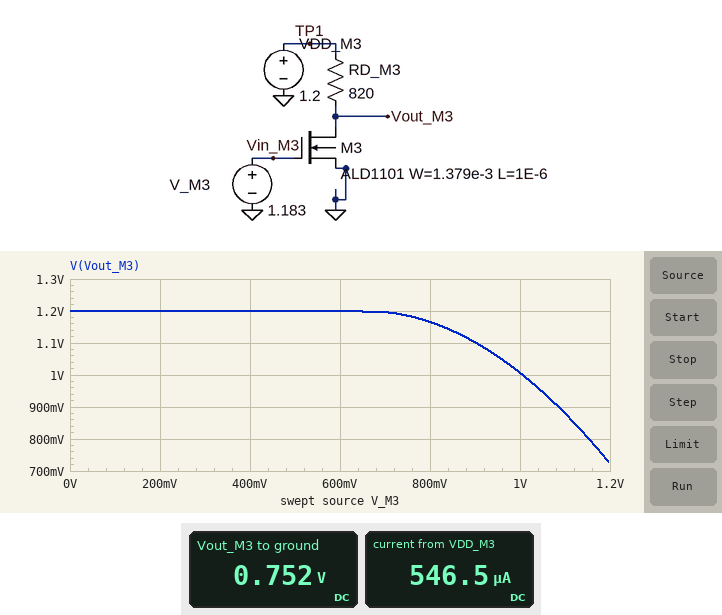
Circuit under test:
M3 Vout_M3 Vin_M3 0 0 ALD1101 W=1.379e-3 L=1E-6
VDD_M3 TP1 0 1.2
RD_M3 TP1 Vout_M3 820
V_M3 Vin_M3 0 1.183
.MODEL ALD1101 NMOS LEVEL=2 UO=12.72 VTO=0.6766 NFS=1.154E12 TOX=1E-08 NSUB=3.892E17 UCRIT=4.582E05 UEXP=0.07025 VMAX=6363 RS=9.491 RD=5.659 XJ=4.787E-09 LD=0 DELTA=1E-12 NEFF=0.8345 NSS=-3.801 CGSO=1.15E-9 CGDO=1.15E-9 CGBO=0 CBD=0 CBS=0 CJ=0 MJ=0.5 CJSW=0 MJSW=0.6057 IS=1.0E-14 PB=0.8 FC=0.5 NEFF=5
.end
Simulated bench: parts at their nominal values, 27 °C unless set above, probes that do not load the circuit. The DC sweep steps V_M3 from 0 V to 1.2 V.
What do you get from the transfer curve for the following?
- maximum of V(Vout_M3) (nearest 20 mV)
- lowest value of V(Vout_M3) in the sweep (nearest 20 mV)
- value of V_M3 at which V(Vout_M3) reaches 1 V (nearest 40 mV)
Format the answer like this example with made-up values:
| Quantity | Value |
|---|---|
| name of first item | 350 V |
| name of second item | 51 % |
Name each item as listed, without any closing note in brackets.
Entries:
| Quantity | Value |
|---|---|
| maximum of V(Vout_M3) | 1.20 V |
| lowest value of V(Vout_M3) in the sweep | 720 mV |
| value of V_M3 at which V(Vout_M3) reaches 1 V | 1.00 V |
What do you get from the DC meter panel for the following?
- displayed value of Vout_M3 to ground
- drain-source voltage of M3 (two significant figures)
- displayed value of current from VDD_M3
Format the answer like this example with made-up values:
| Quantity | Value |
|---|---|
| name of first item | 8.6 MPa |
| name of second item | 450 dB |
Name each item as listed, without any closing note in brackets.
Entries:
| Quantity | Value |
|---|---|
| displayed value of Vout_M3 to ground | 0.752 V |
| drain-source voltage of M3 | 750 mV |
| displayed value of current from VDD_M3 | 546.5 µA |
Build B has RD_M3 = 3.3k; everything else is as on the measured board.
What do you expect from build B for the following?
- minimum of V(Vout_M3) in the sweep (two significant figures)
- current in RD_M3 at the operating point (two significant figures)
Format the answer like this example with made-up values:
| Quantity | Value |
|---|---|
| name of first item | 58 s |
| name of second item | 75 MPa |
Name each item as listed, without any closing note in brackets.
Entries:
| Quantity | Value |
|---|---|
| minimum of V(Vout_M3) in the sweep | 130 mV |
| current in RD_M3 at the operating point | 320 µA |
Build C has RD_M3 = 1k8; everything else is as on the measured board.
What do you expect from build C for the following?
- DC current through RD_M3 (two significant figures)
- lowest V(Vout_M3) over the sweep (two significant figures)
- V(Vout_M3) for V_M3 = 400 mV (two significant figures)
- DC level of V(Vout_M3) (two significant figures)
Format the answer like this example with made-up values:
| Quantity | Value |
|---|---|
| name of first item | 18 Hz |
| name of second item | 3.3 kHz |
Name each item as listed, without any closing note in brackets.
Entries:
| Quantity | Value |
|---|---|
| DC current through RD_M3 | 510 µA |
| lowest V(Vout_M3) over the sweep | 260 mV |
| V(Vout_M3) for V_M3 = 400 mV | 1.2 V |
| DC level of V(Vout_M3) | 280 mV |
